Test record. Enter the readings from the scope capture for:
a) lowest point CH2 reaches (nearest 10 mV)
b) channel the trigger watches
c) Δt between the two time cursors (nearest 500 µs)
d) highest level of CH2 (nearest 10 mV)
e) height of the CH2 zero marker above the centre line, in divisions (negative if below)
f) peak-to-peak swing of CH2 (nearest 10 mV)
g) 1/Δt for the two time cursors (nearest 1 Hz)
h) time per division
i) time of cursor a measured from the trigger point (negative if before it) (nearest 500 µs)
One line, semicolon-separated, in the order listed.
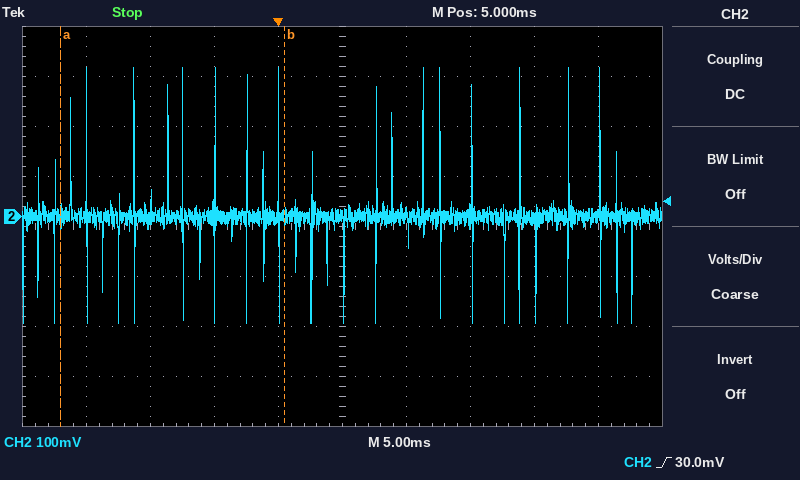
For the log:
-210 mV; CH2; 17.5 ms; 300 mV; +0.2 div; 510 mV; 57 Hz; 5 ms; -17.0 ms
